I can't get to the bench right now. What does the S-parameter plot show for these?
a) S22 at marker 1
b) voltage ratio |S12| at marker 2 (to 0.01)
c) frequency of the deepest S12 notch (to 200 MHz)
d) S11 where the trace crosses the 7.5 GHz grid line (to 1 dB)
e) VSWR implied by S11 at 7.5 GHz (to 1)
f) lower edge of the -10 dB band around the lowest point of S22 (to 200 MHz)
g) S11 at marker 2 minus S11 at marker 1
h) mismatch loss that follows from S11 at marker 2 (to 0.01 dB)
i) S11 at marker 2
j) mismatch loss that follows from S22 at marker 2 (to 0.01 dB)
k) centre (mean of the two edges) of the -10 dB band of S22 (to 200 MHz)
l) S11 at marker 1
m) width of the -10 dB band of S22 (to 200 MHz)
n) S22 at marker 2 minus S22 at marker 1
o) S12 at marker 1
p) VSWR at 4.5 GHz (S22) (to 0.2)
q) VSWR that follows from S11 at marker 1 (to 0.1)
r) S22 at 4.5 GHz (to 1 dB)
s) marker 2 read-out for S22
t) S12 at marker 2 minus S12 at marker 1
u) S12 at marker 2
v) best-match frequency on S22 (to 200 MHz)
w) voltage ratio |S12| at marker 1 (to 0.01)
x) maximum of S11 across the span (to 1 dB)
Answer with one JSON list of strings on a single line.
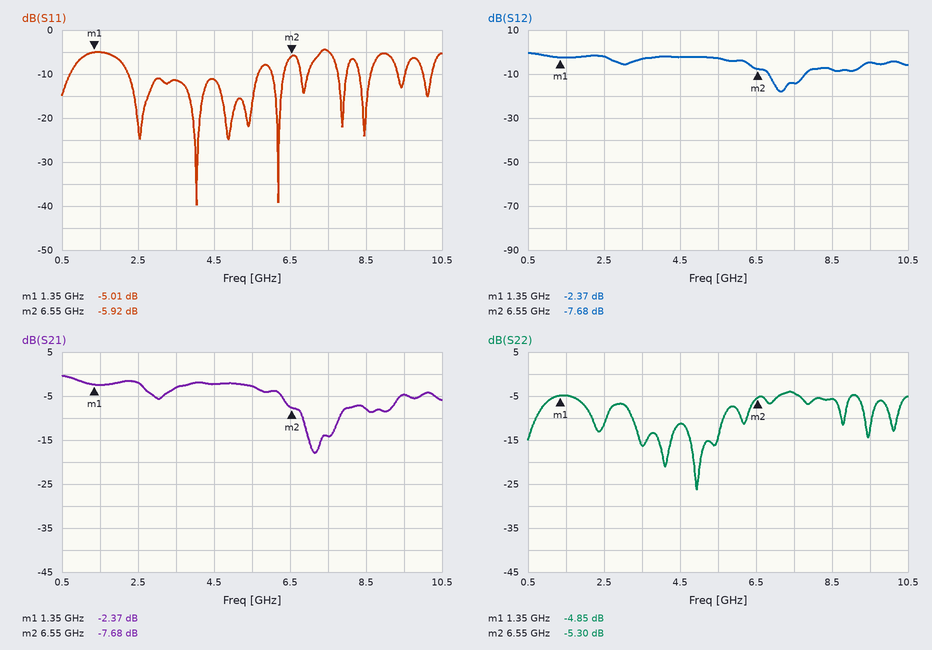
["-4.85 dB", "0.41", "7.2 GHz", "-5 dB", "4", "3.2 GHz", "-0.91 dB", "1.28 dB", "-5.92 dB", "1.52 dB", "4.4 GHz", "-5.01 dB", "2.4 GHz", "-0.45 dB", "-2.37 dB", "1.8", "3.6", "-11 dB", "-5.30 dB", "-5.31 dB", "-7.68 dB", "5.0 GHz", "0.76", "-4 dB"]
